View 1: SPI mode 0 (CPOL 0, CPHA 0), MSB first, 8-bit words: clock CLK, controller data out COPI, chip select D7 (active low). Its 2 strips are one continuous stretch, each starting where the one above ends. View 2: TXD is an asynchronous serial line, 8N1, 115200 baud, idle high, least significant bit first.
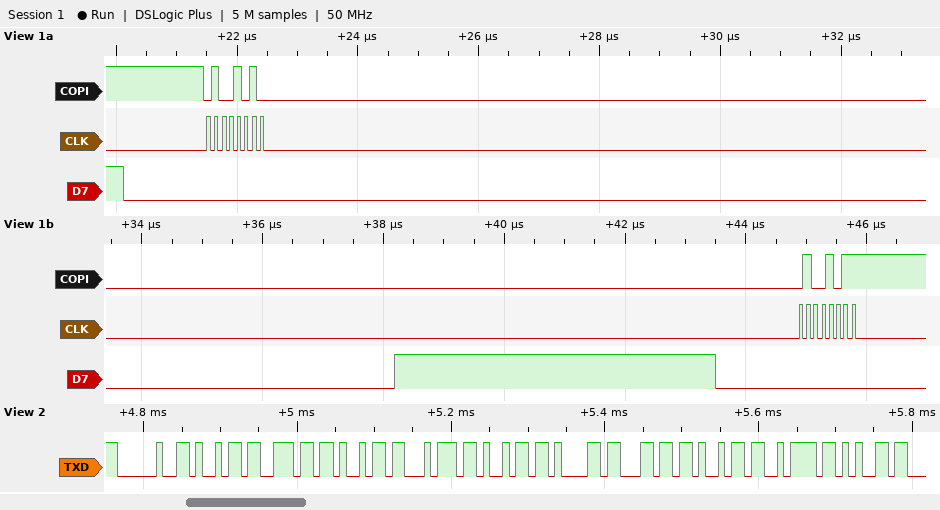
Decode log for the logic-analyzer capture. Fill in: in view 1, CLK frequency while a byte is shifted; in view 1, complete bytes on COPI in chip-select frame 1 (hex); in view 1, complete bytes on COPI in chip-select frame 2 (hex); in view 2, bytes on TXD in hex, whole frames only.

8 MHz
0x4A
0x4B
20 69 6E 69 74 69 61 6C 69 7A 65
